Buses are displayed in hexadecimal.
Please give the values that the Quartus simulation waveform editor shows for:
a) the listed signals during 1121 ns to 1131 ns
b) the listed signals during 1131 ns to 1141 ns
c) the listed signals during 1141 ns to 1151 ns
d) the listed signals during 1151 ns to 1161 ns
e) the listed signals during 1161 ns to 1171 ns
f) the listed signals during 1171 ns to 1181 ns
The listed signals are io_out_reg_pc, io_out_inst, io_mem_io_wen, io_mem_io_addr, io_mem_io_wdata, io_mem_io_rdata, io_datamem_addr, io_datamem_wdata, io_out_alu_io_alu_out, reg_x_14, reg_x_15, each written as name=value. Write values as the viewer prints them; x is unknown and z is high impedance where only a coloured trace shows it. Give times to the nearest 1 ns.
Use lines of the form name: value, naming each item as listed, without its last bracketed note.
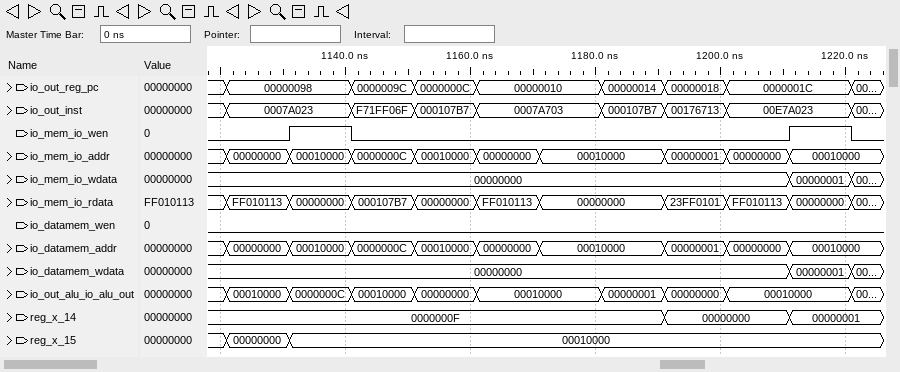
the listed signals during 1121 ns to 1131 ns: io_out_reg_pc=00000098, io_out_inst=0007A023, io_mem_io_wen=0, io_mem_io_addr=00000000, io_mem_io_wdata=00000000, io_mem_io_rdata=FF010113, io_datamem_addr=00000000, io_datamem_wdata=00000000, io_out_alu_io_alu_out=00010000, reg_x_14=0000000F, reg_x_15=00000000
the listed signals during 1131 ns to 1141 ns: io_out_reg_pc=00000098, io_out_inst=0007A023, io_mem_io_wen=1, io_mem_io_addr=00010000, io_mem_io_wdata=00000000, io_mem_io_rdata=00000000, io_datamem_addr=00010000, io_datamem_wdata=00000000, io_out_alu_io_alu_out=0000000C, reg_x_14=0000000F, reg_x_15=00010000
the listed signals during 1141 ns to 1151 ns: io_out_reg_pc=0000009C, io_out_inst=F71FF06F, io_mem_io_wen=0, io_mem_io_addr=0000000C, io_mem_io_wdata=00000000, io_mem_io_rdata=000107B7, io_datamem_addr=0000000C, io_datamem_wdata=00000000, io_out_alu_io_alu_out=00010000, reg_x_14=0000000F, reg_x_15=00010000
the listed signals during 1151 ns to 1161 ns: io_out_reg_pc=0000000C, io_out_inst=000107B7, io_mem_io_wen=0, io_mem_io_addr=00010000, io_mem_io_wdata=00000000, io_mem_io_rdata=00000000, io_datamem_addr=00010000, io_datamem_wdata=00000000, io_out_alu_io_alu_out=00000000, reg_x_14=0000000F, reg_x_15=00010000
the listed signals during 1161 ns to 1171 ns: io_out_reg_pc=00000010, io_out_inst=0007A703, io_mem_io_wen=0, io_mem_io_addr=00000000, io_mem_io_wdata=00000000, io_mem_io_rdata=FF010113, io_datamem_addr=00000000, io_datamem_wdata=00000000, io_out_alu_io_alu_out=00010000, reg_x_14=0000000F, reg_x_15=00010000
the listed signals during 1171 ns to 1181 ns: io_out_reg_pc=00000010, io_out_inst=0007A703, io_mem_io_wen=0, io_mem_io_addr=00010000, io_mem_io_wdata=00000000, io_mem_io_rdata=00000000, io_datamem_addr=00010000, io_datamem_wdata=00000000, io_out_alu_io_alu_out=00010000, reg_x_14=0000000F, reg_x_15=00010000
